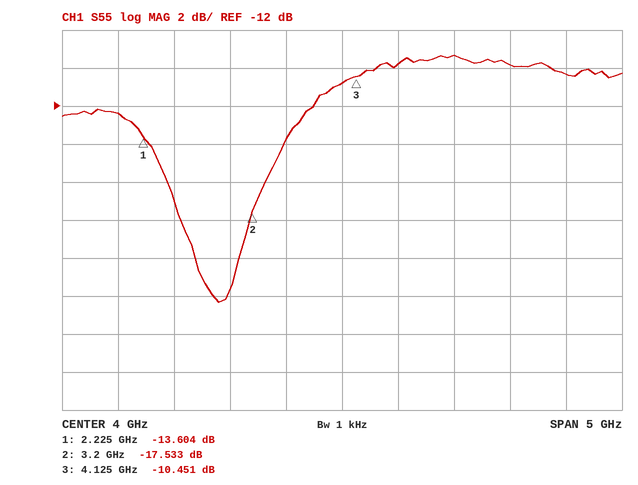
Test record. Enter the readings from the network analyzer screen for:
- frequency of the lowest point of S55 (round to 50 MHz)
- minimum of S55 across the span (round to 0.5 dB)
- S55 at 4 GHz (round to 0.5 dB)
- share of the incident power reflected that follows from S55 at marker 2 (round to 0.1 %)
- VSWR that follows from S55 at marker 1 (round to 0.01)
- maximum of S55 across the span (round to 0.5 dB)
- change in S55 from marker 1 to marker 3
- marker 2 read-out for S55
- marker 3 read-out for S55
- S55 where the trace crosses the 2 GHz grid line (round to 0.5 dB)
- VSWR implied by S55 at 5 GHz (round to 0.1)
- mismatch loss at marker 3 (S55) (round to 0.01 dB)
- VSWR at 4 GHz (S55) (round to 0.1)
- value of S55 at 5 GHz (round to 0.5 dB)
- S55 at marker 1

2.90 GHz
-22.5 dB
-11.0 dB
1.8 %
1.53
-9.5 dB
3.153 dB
-17.533 dB
-10.451 dB
-12.5 dB
2.0
0.41 dB
1.8
-9.5 dB
-13.604 dB
